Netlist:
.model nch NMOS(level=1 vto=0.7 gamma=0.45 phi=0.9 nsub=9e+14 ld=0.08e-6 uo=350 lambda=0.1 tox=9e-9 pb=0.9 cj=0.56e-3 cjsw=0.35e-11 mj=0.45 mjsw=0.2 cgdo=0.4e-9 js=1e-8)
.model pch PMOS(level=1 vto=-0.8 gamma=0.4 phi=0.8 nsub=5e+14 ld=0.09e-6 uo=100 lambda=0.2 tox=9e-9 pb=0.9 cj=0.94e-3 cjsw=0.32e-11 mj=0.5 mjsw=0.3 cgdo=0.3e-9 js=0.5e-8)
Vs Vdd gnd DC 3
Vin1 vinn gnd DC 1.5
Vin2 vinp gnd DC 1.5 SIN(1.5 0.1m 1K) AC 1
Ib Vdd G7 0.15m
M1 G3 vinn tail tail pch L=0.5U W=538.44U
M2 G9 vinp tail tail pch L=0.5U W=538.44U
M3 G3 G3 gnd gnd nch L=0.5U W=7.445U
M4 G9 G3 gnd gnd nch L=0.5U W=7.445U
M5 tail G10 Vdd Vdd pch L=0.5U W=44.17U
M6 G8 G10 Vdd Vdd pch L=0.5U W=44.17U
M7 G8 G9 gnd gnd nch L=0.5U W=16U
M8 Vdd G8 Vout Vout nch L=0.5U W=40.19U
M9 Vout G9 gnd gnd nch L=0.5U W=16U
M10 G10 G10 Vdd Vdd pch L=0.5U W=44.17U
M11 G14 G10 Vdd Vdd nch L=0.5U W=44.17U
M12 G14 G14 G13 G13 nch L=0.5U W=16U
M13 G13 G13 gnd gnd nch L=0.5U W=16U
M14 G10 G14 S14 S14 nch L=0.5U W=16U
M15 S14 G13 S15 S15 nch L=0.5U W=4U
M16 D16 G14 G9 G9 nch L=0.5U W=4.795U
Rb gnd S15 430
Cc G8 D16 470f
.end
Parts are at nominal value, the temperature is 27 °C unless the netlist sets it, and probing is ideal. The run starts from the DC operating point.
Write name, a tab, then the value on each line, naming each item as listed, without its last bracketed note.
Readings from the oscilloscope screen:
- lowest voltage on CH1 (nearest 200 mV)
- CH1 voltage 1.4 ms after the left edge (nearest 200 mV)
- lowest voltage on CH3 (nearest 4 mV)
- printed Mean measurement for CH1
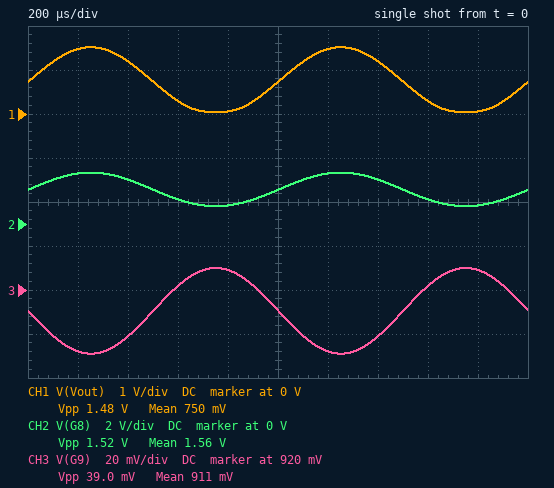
lowest voltage on CH1	0 V
CH1 voltage 1.4 ms after the left edge	1.2 V
lowest voltage on CH3	892 mV
printed Mean measurement for CH1	750 mV
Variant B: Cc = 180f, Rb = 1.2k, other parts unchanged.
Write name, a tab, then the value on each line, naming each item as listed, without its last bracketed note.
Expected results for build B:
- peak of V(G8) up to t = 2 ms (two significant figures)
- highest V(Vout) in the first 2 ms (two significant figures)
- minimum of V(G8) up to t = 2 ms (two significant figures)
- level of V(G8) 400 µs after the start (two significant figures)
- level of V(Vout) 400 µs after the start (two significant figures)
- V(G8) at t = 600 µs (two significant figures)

peak of V(G8) up to t = 2 ms	2.6 V
highest V(Vout) in the first 2 ms	1.8 V
minimum of V(G8) up to t = 2 ms	500 mV
level of V(G8) 400 µs after the start	2.2 V
level of V(Vout) 400 µs after the start	1.4 V
V(G8) at t = 600 µs	930 mV
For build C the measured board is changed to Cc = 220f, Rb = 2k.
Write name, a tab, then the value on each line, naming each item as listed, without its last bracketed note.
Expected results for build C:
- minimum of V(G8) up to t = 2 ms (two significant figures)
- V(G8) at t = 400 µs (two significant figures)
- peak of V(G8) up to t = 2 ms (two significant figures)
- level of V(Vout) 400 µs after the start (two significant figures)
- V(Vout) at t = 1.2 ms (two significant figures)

minimum of V(G8) up to t = 2 ms	220 mV
V(G8) at t = 400 µs	2.4 V
peak of V(G8) up to t = 2 ms	2.9 V
level of V(Vout) 400 µs after the start	1.6 V
V(Vout) at t = 1.2 ms	2.1 V
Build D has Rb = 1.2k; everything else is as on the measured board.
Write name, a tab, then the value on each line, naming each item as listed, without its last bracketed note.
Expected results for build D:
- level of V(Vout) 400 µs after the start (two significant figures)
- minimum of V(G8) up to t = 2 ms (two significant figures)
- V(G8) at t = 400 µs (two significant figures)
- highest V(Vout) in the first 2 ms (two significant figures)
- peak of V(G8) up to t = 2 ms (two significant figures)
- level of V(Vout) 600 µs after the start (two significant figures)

level of V(Vout) 400 µs after the start	1.4 V
minimum of V(G8) up to t = 2 ms	500 mV
V(G8) at t = 400 µs	2.2 V
highest V(Vout) in the first 2 ms	1.8 V
peak of V(G8) up to t = 2 ms	2.6 V
level of V(Vout) 600 µs after the start	130 mV
